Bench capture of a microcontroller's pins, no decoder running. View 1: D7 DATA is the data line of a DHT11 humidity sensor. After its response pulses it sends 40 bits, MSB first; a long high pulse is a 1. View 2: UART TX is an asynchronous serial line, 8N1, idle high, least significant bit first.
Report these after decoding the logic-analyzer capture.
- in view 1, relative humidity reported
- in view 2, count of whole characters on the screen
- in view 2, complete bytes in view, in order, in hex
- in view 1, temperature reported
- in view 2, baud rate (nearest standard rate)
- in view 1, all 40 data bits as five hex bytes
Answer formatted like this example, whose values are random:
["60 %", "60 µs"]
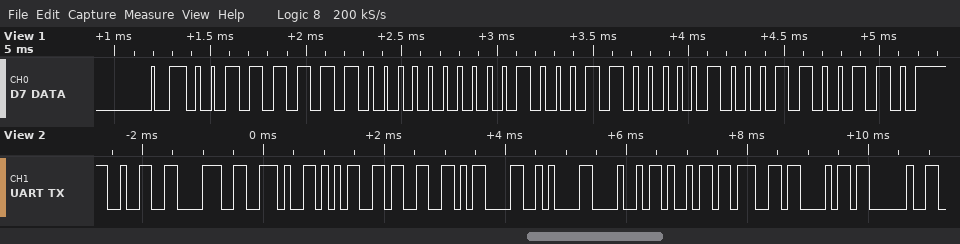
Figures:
["63 %", "12", "32 38 2E 35 33 0D 0A 48 69 67 68 20", "35.4 °C", "9600 baud", "3F 00 23 04 66"]
